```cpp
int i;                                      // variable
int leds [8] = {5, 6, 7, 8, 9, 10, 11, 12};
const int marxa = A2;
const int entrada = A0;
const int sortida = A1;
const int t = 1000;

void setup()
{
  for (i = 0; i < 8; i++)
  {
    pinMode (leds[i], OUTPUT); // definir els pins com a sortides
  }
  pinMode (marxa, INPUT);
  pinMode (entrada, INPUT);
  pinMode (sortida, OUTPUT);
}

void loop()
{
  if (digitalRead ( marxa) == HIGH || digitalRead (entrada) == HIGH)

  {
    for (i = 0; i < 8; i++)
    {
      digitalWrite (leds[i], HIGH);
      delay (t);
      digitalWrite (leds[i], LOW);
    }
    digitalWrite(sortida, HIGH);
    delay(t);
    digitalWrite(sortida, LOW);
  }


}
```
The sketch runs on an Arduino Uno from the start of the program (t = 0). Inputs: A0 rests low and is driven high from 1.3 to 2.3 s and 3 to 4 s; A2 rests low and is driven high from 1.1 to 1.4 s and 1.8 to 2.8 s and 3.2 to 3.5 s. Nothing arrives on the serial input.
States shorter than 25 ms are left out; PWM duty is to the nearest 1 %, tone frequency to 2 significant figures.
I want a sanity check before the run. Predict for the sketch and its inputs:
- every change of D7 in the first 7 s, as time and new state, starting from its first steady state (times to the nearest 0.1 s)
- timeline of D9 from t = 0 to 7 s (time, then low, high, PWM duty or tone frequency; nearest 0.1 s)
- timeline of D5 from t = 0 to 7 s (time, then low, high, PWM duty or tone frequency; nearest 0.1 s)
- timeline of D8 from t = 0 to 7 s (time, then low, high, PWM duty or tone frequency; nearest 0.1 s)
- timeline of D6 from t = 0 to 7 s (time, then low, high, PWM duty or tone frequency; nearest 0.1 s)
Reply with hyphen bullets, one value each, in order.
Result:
- 0 s low; 3.1 s high; 4.1 s low
- 0 s low; 5.1 s high; 6.1 s low
- 0 s low; 1.1 s high; 2.1 s low
- 0 s low; 4.1 s high; 5.1 s low
- 0 s low; 2.1 s high; 3.1 s low
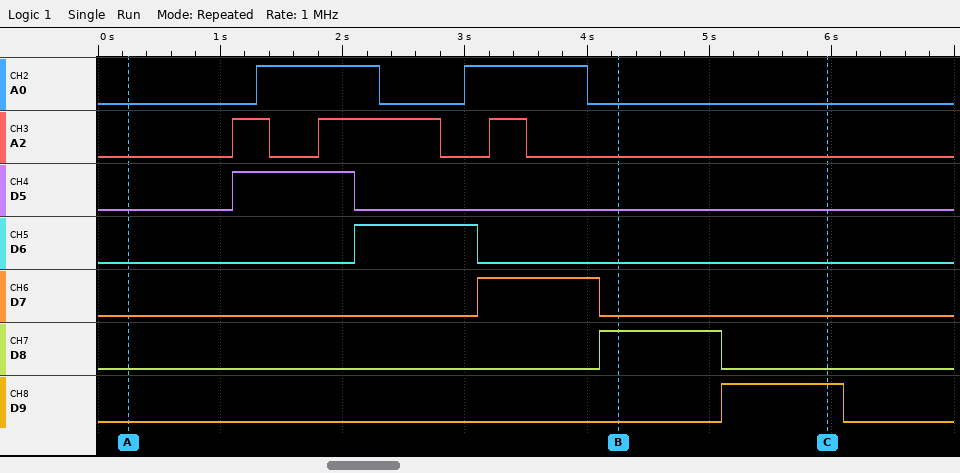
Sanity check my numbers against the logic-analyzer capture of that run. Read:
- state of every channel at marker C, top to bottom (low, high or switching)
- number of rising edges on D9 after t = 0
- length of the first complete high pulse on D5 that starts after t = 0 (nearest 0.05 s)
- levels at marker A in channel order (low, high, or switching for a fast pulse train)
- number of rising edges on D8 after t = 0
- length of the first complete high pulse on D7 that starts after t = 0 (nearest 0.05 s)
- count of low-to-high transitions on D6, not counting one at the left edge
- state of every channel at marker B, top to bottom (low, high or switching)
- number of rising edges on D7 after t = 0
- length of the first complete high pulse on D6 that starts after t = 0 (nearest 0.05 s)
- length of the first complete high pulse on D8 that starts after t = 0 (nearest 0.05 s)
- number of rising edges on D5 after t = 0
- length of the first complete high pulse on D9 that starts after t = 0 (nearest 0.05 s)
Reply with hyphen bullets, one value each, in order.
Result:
- A0 low, A2 low, D5 low, D6 low, D7 low, D8 low, D9 high
- 1
- 1.00 s
- A0 low, A2 low, D5 low, D6 low, D7 low, D8 low, D9 low
- 1
- 1.00 s
- 1
- A0 low, A2 low, D5 low, D6 low, D7 low, D8 high, D9 low
- 1
- 1.00 s
- 1.00 s
- 1
- 1.00 s
